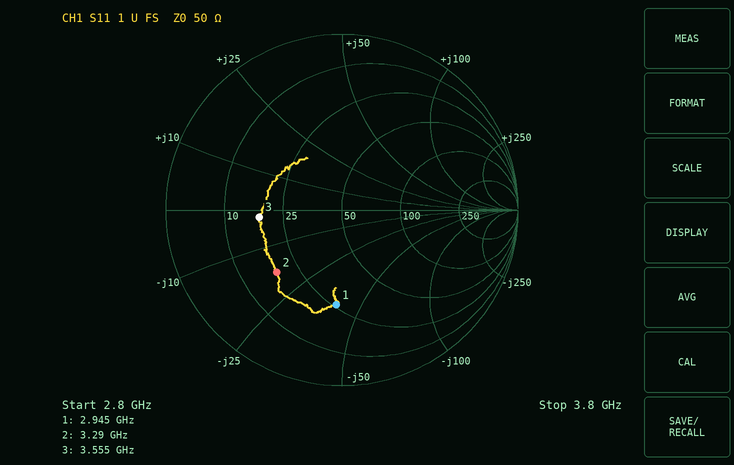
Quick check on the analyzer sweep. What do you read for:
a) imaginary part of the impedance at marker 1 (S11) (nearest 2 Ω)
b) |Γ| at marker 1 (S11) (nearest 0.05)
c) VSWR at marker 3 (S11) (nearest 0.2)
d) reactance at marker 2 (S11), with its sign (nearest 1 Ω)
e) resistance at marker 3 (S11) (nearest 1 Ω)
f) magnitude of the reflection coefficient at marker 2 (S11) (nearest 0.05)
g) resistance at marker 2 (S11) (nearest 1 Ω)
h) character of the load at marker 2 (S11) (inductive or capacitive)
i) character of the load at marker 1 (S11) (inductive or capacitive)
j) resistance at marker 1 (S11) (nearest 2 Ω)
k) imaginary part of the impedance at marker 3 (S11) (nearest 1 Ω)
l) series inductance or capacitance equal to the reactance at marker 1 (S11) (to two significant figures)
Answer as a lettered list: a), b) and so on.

a) -40 Ω
b) 0.55
c) 2.8
d) -18 Ω
e) 18 Ω
f) 0.50
g) 18 Ω
h) capacitive
i) capacitive
j) 26 Ω
k) -2 Ω
l) 1.4 pF
